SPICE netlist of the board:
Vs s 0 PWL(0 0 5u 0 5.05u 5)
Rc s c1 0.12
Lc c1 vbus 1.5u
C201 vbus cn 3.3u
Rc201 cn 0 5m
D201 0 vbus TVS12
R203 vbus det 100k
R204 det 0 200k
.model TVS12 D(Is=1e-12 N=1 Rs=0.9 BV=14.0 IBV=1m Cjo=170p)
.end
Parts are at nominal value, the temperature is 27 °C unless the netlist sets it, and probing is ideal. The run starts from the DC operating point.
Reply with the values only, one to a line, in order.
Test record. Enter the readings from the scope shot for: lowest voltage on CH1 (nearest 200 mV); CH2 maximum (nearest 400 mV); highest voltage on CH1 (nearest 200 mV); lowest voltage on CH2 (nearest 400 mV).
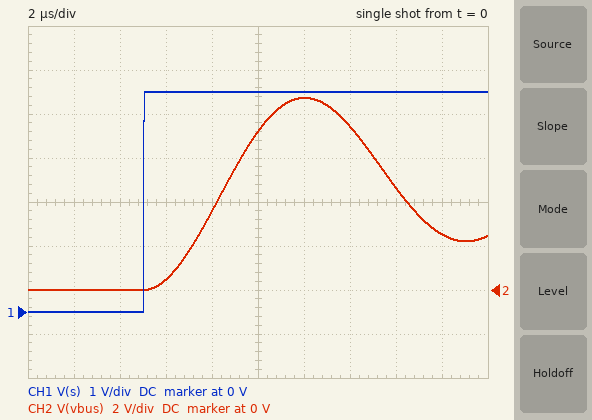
0 V
8.8 V
5.0 V
0 V
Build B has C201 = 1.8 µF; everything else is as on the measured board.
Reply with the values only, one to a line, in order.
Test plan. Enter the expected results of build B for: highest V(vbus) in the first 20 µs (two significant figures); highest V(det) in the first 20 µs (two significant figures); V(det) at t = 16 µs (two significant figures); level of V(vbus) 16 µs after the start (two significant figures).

9.0 V
6.0 V
1.3 V
2.0 V
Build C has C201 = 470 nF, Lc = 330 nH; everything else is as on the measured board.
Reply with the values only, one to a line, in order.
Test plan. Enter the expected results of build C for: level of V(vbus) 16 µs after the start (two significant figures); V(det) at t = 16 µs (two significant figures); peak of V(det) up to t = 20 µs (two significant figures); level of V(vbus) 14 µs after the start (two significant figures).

5.5 V
3.7 V
6.0 V
5.7 V
